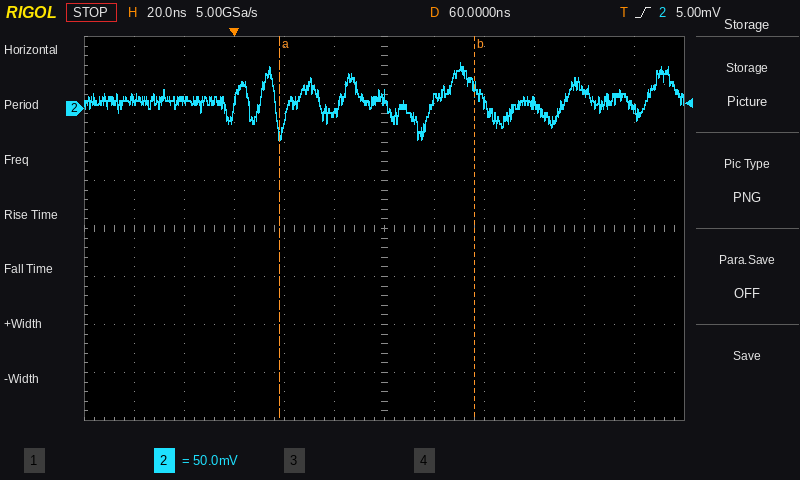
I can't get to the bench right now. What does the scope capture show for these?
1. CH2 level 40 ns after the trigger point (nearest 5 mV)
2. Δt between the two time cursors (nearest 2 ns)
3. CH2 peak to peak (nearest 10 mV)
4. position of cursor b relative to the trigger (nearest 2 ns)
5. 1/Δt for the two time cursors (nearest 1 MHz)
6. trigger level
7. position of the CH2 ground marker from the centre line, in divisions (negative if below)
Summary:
-5 mV
78 ns
80 mV
+96 ns
13 MHz
5.00 mV
+2.5 div
